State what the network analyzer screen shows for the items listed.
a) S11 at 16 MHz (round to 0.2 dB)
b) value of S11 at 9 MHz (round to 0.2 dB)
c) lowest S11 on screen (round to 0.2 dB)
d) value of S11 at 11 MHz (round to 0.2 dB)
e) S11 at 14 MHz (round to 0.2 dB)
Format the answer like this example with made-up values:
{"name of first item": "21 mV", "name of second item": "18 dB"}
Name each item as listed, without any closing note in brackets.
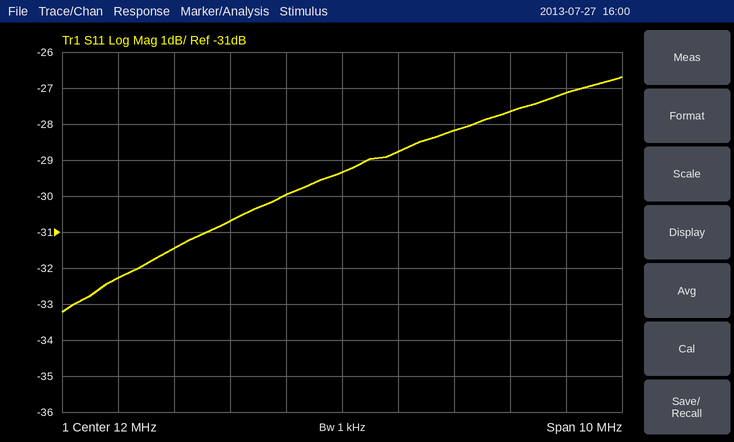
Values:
{"S11 at 16 MHz": "-27.2 dB", "value of S11 at 9 MHz": "-31.4 dB", "lowest S11 on screen": "-33.2 dB", "value of S11 at 11 MHz": "-30.0 dB", "S11 at 14 MHz": "-28.2 dB"}
